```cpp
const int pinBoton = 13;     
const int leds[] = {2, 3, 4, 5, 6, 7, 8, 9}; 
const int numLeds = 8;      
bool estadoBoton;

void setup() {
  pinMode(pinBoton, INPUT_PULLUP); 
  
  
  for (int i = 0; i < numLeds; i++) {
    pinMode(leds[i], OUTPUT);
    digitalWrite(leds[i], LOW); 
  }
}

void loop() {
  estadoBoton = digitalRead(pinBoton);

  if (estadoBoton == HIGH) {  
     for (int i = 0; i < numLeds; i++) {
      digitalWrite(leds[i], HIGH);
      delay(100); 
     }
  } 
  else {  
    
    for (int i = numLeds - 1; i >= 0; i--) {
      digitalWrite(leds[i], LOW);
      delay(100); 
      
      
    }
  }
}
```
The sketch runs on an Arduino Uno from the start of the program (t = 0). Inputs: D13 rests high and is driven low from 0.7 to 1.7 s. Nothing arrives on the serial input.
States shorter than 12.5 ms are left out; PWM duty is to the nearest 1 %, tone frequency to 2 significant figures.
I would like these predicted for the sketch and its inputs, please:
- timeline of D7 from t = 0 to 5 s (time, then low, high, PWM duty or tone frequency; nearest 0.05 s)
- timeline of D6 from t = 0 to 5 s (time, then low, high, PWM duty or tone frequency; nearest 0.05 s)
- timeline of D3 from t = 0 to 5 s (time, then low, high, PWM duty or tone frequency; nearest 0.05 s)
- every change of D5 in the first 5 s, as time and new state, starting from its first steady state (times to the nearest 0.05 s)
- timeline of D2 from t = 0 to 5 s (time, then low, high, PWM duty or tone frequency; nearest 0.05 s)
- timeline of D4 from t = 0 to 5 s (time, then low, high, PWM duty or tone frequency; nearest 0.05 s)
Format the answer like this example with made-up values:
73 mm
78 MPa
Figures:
0 s low; 0.5 s high; 1 s low; 2.9 s high
0 s low; 0.4 s high; 1.1 s low; 2.8 s high
0 s low; 0.1 s high; 1.4 s low; 2.5 s high
0 s low; 0.3 s high; 1.2 s low; 2.7 s high
0 s high; 1.5 s low; 2.4 s high
0 s low; 0.2 s high; 1.3 s low; 2.6 s high
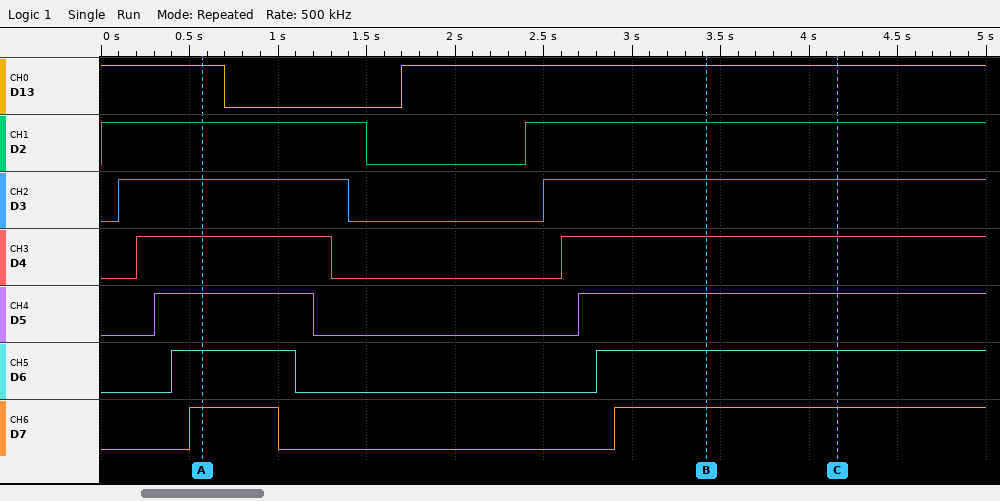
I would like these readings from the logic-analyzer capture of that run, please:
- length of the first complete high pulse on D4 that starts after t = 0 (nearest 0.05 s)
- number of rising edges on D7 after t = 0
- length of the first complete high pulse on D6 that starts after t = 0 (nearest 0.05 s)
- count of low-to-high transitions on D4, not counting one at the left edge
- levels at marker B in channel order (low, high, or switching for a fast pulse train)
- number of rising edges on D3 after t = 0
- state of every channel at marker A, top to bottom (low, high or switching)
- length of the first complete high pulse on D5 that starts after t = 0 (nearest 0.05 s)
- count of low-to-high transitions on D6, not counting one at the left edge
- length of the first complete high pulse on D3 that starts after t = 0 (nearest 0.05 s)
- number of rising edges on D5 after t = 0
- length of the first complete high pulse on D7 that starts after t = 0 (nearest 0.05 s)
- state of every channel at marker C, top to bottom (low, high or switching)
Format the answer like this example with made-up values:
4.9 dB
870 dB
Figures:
1.10 s
2
0.70 s
2
D13 high, D2 high, D3 high, D4 high, D5 high, D6 high, D7 high
2
D13 high, D2 high, D3 high, D4 high, D5 high, D6 high, D7 high
0.90 s
2
1.30 s
2
0.50 s
D13 high, D2 high, D3 high, D4 high, D5 high, D6 high, D7 high
